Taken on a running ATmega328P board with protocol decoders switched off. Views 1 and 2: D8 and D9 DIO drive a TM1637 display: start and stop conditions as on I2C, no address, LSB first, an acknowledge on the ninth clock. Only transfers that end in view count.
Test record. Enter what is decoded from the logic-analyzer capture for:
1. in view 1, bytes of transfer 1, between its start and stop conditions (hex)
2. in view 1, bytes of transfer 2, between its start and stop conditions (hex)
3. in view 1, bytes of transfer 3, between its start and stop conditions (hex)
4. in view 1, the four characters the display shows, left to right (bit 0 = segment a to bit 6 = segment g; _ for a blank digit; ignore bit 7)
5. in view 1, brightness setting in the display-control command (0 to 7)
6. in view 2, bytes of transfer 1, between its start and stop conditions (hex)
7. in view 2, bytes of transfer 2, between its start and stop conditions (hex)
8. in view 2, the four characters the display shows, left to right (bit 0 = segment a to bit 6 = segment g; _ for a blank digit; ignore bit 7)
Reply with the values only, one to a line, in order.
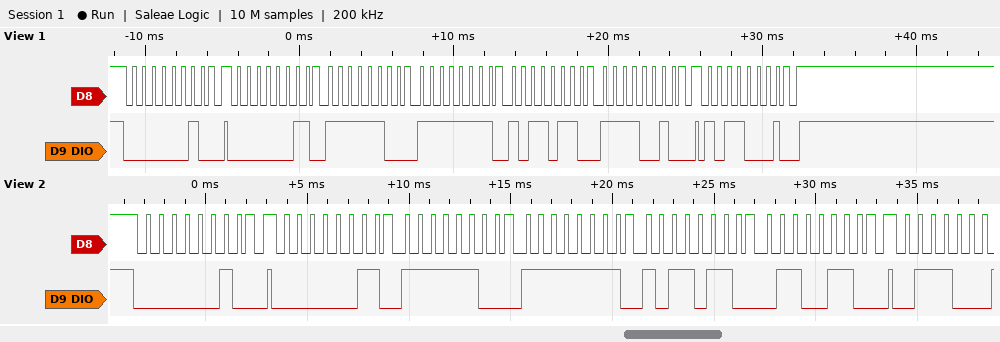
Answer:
40
C0 3F FF 6D 4F
8D
0853
5
40
C0 3F FF 6D 66
0854
